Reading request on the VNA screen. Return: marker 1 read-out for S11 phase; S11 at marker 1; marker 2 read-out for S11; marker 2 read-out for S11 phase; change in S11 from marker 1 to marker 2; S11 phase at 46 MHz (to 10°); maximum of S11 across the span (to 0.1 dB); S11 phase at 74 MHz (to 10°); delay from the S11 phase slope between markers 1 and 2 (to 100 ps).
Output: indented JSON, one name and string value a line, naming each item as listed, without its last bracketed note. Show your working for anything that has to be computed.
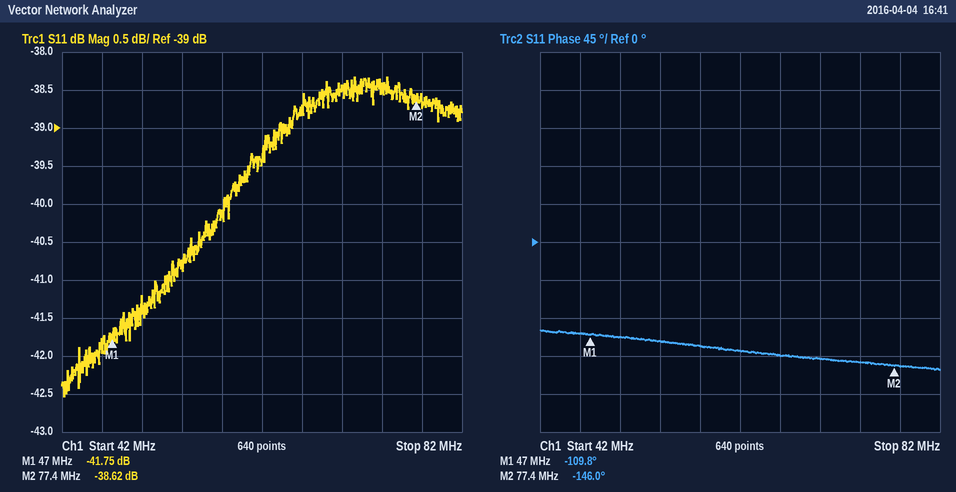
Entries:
{
  "marker 1 read-out for S11 phase": "-109.8°",
  "S11 at marker 1": "-41.75 dB",
  "marker 2 read-out for S11": "-38.62 dB",
  "marker 2 read-out for S11 phase": "-146.0°",
  "change in S11 from marker 1 to marker 2": "-38.62 − (-41.75) = 3.13 dB",
  "S11 phase at 46 MHz": "-110°",
  "maximum of S11 across the span": "-38.3 dB",
  "S11 phase at 74 MHz": "-140°",
  "delay from the S11 phase slope between markers 1 and 2": "−(-146° − (-109.8°))/(360° × 30.4 MHz) ≈ 3.3 ns"
}
